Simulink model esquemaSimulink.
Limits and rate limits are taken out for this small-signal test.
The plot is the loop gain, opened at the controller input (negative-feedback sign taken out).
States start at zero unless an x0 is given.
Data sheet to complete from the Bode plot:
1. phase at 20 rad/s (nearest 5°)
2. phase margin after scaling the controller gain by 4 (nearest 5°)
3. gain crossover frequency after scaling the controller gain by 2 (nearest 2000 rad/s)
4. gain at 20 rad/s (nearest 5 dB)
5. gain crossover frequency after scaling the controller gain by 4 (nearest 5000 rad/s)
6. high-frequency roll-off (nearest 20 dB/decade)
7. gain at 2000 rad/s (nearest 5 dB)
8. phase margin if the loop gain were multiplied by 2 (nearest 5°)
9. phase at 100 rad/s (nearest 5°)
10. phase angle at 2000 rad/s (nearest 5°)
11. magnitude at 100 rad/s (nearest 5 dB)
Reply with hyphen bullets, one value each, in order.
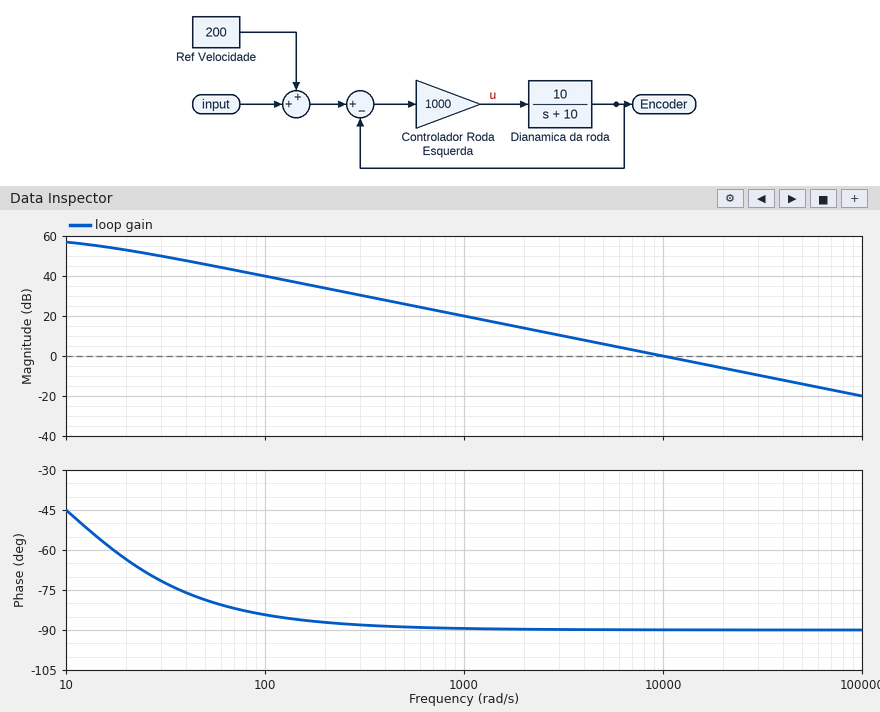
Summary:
- -65°
- 90°
- 20000 rad/s
- 55 dB
- 40000 rad/s
- -20 dB/decade
- 15 dB
- 90°
- -85°
- -90°
- 40 dB
